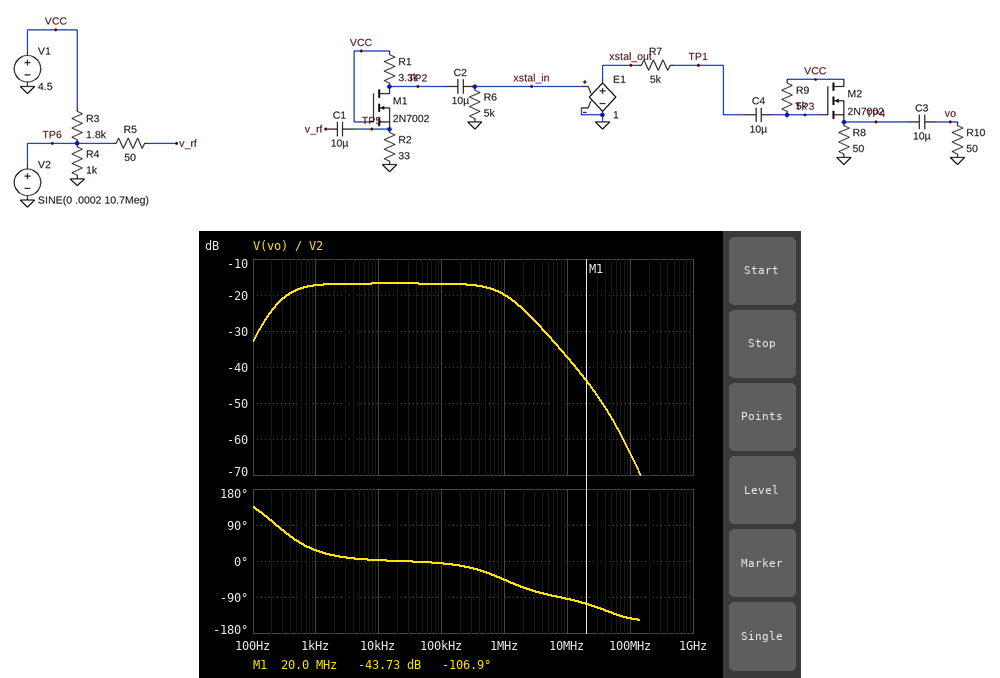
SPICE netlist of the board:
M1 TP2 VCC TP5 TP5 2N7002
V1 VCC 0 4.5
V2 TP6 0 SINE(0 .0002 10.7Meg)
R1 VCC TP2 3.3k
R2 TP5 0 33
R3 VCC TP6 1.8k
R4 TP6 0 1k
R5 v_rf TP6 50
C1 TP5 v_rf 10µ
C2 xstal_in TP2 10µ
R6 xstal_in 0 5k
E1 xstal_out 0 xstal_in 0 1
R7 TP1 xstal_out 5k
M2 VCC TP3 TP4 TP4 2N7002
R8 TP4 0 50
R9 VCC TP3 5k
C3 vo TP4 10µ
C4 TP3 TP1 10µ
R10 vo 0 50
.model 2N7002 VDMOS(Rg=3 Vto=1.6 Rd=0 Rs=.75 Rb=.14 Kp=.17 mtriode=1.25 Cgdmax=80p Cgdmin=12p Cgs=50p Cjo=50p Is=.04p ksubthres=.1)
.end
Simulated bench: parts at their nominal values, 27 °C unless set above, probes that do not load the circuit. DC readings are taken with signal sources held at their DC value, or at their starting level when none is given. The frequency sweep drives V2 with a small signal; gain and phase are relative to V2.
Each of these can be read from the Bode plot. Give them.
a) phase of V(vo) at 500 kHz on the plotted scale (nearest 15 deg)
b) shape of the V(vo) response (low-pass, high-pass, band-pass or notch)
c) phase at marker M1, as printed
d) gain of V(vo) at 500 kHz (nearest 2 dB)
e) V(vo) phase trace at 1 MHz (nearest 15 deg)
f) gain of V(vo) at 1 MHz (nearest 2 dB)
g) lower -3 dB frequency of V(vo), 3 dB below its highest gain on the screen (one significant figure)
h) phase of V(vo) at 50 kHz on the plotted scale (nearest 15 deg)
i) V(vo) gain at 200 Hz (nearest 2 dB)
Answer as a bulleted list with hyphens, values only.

- -30 deg
- band-pass
- -106.9 deg
- -18 dB
- -45 deg
- -20 dB
- 400 Hz
- 0 deg
- -24 dB
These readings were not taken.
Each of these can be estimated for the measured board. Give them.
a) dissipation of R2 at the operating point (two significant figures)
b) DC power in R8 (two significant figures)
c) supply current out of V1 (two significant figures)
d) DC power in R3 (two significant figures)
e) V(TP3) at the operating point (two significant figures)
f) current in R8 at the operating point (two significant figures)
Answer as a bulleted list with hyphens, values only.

- 60 µW
- 93 mW
- 47 mA
- 11 mW
- 4.5 V
- 43 mA
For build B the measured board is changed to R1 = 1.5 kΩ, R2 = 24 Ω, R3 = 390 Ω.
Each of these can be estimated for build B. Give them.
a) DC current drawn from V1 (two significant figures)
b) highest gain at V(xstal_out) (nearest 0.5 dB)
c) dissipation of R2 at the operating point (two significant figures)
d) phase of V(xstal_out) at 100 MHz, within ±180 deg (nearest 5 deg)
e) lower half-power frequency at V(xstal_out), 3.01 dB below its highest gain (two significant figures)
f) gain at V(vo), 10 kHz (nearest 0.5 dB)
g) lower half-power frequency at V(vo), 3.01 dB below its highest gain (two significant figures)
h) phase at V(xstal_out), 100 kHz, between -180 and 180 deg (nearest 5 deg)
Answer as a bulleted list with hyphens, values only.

- 58 mA
- -10.0 dB
- 210 µW
- -45 deg
- 220 Hz
- -18.5 dB
- 380 Hz
- 0 deg
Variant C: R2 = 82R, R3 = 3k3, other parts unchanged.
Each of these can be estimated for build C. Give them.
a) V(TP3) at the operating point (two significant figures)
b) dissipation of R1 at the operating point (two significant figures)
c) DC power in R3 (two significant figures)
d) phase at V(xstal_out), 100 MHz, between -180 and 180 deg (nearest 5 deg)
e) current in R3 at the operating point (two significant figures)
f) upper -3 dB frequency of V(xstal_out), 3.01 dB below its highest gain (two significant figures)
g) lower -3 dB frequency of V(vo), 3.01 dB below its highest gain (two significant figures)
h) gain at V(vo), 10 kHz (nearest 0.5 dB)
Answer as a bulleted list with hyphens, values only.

- 4.5 V
- 5.8 mW
- 6.1 mW
- -60 deg
- 1.4 mA
- 35 MHz
- 320 Hz
- -13.0 dB
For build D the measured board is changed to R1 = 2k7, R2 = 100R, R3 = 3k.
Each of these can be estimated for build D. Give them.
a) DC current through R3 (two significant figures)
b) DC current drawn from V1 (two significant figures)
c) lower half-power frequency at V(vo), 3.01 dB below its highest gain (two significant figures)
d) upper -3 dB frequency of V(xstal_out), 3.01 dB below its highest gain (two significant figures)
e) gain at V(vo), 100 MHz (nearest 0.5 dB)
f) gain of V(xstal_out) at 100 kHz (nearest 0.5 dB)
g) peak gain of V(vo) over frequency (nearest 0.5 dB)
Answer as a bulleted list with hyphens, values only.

- 1.5 mA
- 46 mA
- 310 Hz
- 33 MHz
- -62.5 dB
- -3.5 dB
- -12.5 dB
